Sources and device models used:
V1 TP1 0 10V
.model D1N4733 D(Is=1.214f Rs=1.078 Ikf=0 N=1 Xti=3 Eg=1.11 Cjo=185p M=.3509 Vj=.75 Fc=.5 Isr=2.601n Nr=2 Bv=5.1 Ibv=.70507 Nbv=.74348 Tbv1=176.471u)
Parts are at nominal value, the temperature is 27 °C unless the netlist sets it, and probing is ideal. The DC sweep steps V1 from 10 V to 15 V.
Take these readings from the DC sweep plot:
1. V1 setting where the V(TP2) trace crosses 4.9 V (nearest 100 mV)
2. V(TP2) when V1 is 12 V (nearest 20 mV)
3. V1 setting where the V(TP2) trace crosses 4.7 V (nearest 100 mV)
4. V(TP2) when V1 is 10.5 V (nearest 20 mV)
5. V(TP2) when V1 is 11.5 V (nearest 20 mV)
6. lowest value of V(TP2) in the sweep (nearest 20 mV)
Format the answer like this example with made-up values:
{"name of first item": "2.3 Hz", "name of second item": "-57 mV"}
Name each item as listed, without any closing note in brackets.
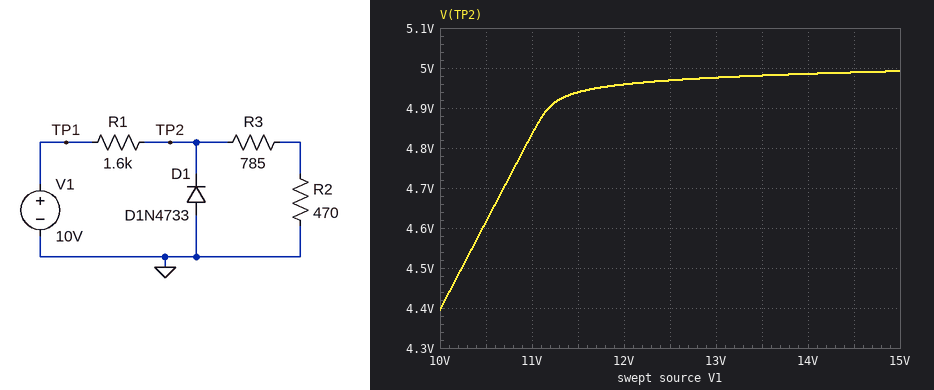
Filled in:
{"V1 setting where the V(TP2) trace crosses 4.9 V": "11.2 V", "V(TP2) when V1 is 12 V": "4.96 V", "V1 setting where the V(TP2) trace crosses 4.7 V": "10.7 V", "V(TP2) when V1 is 10.5 V": "4.62 V", "V(TP2) when V1 is 11.5 V": "4.94 V", "lowest value of V(TP2) in the sweep": "4.40 V"}
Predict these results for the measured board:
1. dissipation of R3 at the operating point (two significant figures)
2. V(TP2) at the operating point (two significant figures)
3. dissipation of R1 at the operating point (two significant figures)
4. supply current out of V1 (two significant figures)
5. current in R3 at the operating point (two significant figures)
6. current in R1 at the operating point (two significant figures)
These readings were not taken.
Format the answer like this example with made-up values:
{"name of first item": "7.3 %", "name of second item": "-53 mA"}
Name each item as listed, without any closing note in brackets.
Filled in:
{"dissipation of R3 at the operating point": "9.6 mW", "V(TP2) at the operating point": "4.4 V", "dissipation of R1 at the operating point": "20 mW", "supply current out of V1": "3.5 mA", "current in R3 at the operating point": "3.5 mA", "current in R1 at the operating point": "3.5 mA"}
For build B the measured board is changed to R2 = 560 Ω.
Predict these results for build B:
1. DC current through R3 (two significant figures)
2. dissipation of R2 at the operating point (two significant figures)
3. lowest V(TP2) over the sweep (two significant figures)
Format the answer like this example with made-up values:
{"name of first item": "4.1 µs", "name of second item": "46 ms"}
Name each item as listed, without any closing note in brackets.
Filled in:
{"DC current through R3": "3.4 mA", "dissipation of R2 at the operating point": "6.5 mW", "lowest V(TP2) over the sweep": "4.6 V"}
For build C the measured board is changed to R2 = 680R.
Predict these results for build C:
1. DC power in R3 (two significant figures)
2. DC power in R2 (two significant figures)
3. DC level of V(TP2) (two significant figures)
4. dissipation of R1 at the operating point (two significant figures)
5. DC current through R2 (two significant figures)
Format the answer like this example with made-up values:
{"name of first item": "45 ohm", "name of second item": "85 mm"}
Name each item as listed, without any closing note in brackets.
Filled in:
{"DC power in R3": "8.4 mW", "DC power in R2": "7.2 mW", "DC level of V(TP2)": "4.8 V", "dissipation of R1 at the operating point": "17 mW", "DC current through R2": "3.3 mA"}
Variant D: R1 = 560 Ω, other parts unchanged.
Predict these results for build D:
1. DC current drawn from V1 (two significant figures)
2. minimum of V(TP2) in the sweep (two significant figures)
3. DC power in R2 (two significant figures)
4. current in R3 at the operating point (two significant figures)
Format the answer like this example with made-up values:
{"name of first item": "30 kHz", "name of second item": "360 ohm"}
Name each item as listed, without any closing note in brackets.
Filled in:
{"DC current drawn from V1": "8.9 mA", "minimum of V(TP2) in the sweep": "5.0 V", "DC power in R2": "7.5 mW", "current in R3 at the operating point": "4.0 mA"}
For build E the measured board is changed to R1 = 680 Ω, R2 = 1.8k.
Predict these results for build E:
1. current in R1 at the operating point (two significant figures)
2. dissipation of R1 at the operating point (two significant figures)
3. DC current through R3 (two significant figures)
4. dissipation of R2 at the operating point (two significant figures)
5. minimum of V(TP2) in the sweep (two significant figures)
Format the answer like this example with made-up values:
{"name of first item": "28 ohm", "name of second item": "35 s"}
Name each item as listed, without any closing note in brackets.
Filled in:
{"current in R1 at the operating point": "7.3 mA", "dissipation of R1 at the operating point": "37 mW", "DC current through R3": "1.9 mA", "dissipation of R2 at the operating point": "6.8 mW", "minimum of V(TP2) in the sweep": "5.0 V"}
